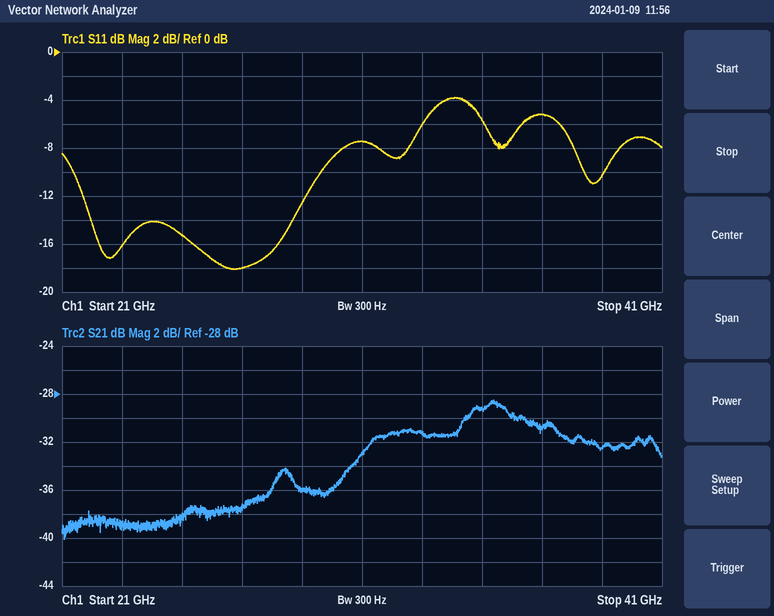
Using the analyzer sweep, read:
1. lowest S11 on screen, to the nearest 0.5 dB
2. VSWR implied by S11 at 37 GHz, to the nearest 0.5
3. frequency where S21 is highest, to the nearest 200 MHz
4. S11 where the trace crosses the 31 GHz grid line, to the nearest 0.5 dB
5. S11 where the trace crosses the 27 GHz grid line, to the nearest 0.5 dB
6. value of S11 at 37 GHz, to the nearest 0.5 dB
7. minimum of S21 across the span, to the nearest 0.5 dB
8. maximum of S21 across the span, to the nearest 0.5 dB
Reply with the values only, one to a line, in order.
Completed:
-18.0 dB
3.5
35.4 GHz
-7.5 dB
-18.0 dB
-5.0 dB
-40.0 dB
-28.5 dB
